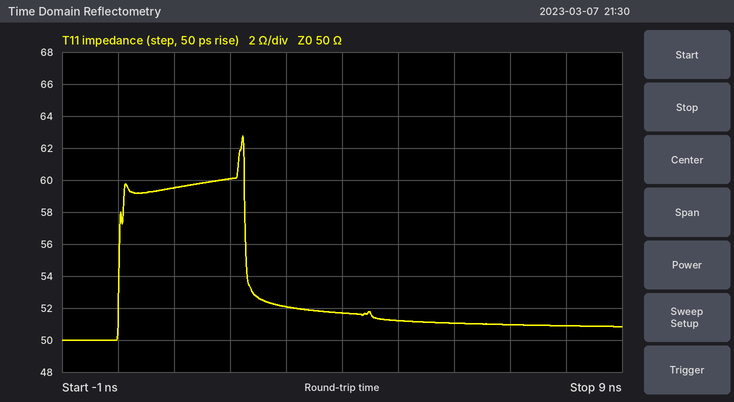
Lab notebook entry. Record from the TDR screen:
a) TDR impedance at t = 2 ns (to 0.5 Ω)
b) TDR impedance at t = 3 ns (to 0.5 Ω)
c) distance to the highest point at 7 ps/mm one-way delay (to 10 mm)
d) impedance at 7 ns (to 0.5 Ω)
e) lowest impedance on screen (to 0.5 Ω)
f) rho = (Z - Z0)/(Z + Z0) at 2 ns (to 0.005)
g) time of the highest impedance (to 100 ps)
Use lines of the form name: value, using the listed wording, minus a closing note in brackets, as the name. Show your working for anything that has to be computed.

TDR impedance at t = 2 ns: 60.0 Ω
TDR impedance at t = 3 ns: 52.0 Ω
distance to the highest point at 7 ps/mm one-way delay: 2.2 ns / 2 / 7 ps/mm ≈ 157 mm, so 160 mm to the nearest 10 mm
impedance at 7 ns: 51.0 Ω
lowest impedance on screen: 50.0 Ω
rho = (Z - Z0)/(Z + Z0) at 2 ns: (60 − 50)/(60 + 50) ≈ +0.0909, so +0.090 to the nearest 0.005
time of the highest impedance: 2.2 ns
